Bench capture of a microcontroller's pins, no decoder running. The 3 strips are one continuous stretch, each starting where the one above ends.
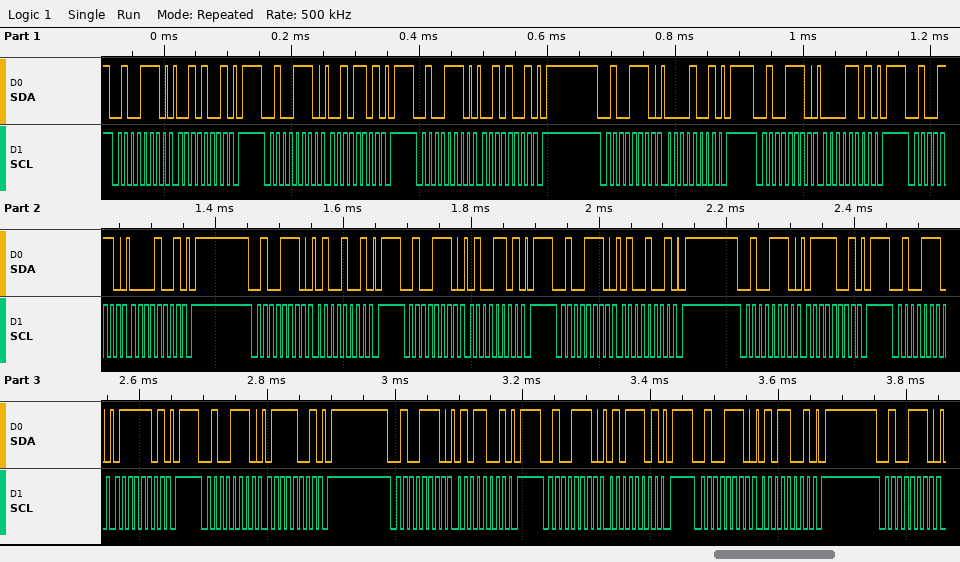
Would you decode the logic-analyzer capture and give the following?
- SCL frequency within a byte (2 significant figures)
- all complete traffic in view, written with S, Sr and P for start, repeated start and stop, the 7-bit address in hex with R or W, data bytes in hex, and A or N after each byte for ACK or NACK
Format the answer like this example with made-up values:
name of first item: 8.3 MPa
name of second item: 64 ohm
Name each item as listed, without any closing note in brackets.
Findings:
SCL frequency within a byte: 100 kHz
all complete traffic in view, written with S, Sr and P for start, repeated start and stop, the 7-bit address in hex with R or W, data bytes in hex, and A or N after each byte for ACK or NACK: S 27W A 29 A P S 27W A 2D A P S 27W A 29 A P S 27W A 09 A P S 27W A 0D A P S 27W A 09 A P S 27W A 49 A P S 27W A 4D A P S 27W A 49 A P S 27W A 79 A P S 27W A 7D A P S 27W A 79 A P S 27W A 59 A P S 27W A 5D A P S 27W A 59 A P S 27W A
